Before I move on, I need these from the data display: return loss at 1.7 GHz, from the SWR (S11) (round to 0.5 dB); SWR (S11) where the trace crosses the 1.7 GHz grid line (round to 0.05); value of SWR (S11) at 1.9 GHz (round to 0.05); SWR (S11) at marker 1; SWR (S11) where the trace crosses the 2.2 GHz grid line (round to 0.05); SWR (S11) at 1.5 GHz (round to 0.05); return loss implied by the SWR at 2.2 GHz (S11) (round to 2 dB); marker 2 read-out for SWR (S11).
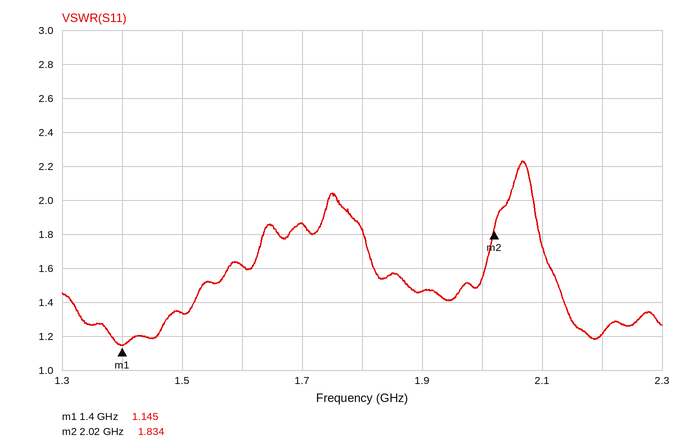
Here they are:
10.5 dB
1.85
1.45
1.145
1.20
1.35
20 dB
1.834
